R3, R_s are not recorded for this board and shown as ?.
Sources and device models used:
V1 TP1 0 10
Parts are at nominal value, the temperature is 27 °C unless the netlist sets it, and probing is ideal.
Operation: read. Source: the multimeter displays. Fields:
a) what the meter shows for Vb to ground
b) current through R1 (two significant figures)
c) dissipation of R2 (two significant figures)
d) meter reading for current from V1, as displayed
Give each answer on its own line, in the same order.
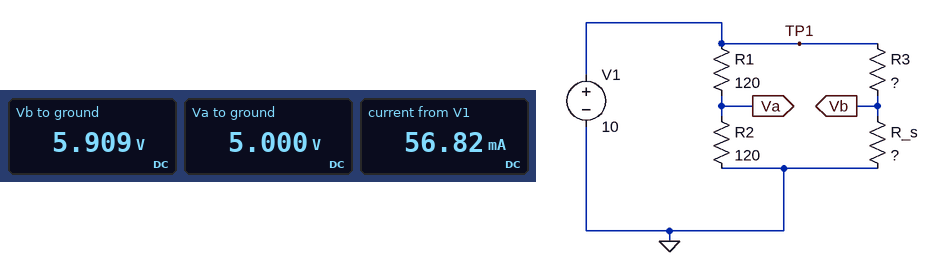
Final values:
5.909 V
42 mA
210 mW
56.82 mA
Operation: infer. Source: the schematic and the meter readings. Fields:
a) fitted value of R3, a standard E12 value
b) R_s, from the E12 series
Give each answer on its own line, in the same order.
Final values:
270 Ω
390 Ω
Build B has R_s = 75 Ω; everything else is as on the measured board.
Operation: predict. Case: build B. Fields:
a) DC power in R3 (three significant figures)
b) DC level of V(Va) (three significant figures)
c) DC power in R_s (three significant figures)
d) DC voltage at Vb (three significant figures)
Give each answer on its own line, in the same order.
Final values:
227 mW
5.00 V
63.0 mW
2.17 V
